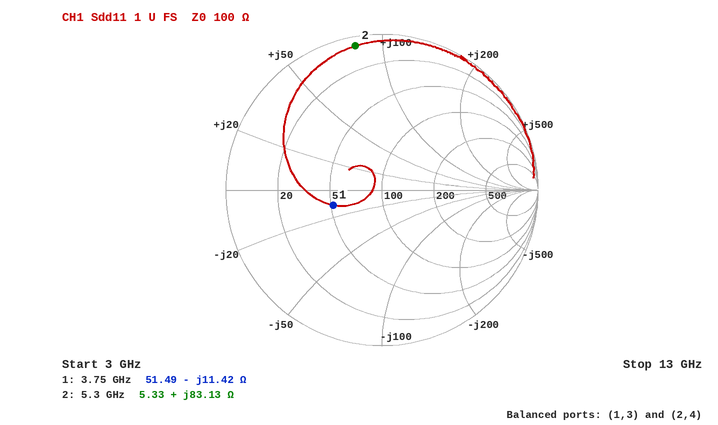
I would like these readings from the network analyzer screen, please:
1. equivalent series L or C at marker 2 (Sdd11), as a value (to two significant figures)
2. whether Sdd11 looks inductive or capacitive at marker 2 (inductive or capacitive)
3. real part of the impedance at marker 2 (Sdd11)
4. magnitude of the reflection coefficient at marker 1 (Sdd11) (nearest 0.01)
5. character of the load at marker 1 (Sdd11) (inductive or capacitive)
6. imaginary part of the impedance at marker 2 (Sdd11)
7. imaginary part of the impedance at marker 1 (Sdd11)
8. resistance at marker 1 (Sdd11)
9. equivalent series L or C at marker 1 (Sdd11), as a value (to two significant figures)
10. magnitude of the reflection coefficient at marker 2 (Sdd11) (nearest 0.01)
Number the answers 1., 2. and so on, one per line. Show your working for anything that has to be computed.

1. L = 83.13 Ω/(2π × 5.3 GHz) ≈ 2.5 nH
2. inductive
3. 5.33 Ω
4. 0.33
5. capacitive
6. +83.13 Ω
7. -11.42 Ω
8. 51.49 Ω
9. C = 1/(2π × 3.75 GHz × 11.42 Ω) ≈ 3.7 pF
10. 0.94
